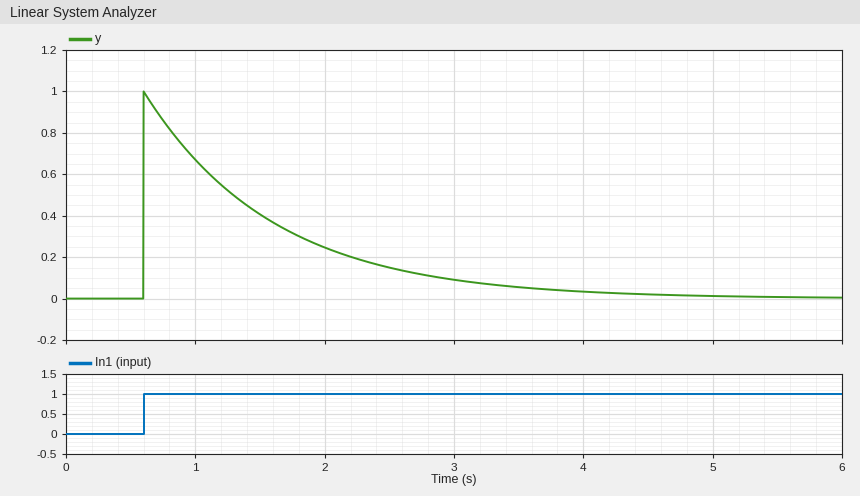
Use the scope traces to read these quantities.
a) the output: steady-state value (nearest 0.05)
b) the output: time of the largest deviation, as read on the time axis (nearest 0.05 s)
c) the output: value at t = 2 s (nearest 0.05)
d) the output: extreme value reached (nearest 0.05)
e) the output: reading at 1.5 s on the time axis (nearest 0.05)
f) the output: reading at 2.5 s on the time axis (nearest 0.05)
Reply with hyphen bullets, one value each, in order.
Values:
- 0.00
- 0.60 s
- 0.25
- 1.00
- 0.40
- 0.15
